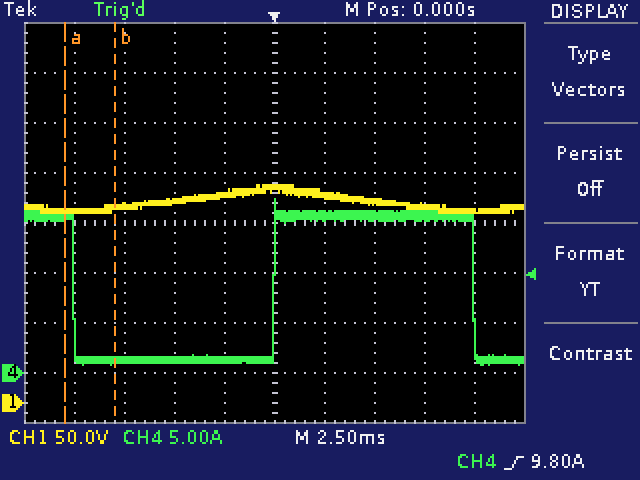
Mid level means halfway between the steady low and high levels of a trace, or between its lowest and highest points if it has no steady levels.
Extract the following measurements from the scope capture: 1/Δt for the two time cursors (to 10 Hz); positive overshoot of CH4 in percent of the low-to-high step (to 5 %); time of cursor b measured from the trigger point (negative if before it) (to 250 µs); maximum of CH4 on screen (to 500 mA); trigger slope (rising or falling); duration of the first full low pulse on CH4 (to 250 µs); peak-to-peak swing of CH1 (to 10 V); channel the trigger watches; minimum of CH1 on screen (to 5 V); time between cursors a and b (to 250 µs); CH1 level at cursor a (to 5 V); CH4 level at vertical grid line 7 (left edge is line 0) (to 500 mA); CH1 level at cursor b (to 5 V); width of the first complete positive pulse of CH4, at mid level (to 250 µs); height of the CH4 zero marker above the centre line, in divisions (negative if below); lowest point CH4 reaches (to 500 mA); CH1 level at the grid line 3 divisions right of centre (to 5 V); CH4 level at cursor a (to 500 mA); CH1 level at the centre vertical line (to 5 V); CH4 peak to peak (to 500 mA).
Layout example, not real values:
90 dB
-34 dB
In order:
400 Hz
10 %
-8.00 ms
17.5 A
rising
10.00 ms
30 V
CH4
190 V
2.50 ms
190 V
15.5 A
195 V
10.00 ms
-3.0 div
1.0 A
195 V
15.5 A
215 V
16.5 A
